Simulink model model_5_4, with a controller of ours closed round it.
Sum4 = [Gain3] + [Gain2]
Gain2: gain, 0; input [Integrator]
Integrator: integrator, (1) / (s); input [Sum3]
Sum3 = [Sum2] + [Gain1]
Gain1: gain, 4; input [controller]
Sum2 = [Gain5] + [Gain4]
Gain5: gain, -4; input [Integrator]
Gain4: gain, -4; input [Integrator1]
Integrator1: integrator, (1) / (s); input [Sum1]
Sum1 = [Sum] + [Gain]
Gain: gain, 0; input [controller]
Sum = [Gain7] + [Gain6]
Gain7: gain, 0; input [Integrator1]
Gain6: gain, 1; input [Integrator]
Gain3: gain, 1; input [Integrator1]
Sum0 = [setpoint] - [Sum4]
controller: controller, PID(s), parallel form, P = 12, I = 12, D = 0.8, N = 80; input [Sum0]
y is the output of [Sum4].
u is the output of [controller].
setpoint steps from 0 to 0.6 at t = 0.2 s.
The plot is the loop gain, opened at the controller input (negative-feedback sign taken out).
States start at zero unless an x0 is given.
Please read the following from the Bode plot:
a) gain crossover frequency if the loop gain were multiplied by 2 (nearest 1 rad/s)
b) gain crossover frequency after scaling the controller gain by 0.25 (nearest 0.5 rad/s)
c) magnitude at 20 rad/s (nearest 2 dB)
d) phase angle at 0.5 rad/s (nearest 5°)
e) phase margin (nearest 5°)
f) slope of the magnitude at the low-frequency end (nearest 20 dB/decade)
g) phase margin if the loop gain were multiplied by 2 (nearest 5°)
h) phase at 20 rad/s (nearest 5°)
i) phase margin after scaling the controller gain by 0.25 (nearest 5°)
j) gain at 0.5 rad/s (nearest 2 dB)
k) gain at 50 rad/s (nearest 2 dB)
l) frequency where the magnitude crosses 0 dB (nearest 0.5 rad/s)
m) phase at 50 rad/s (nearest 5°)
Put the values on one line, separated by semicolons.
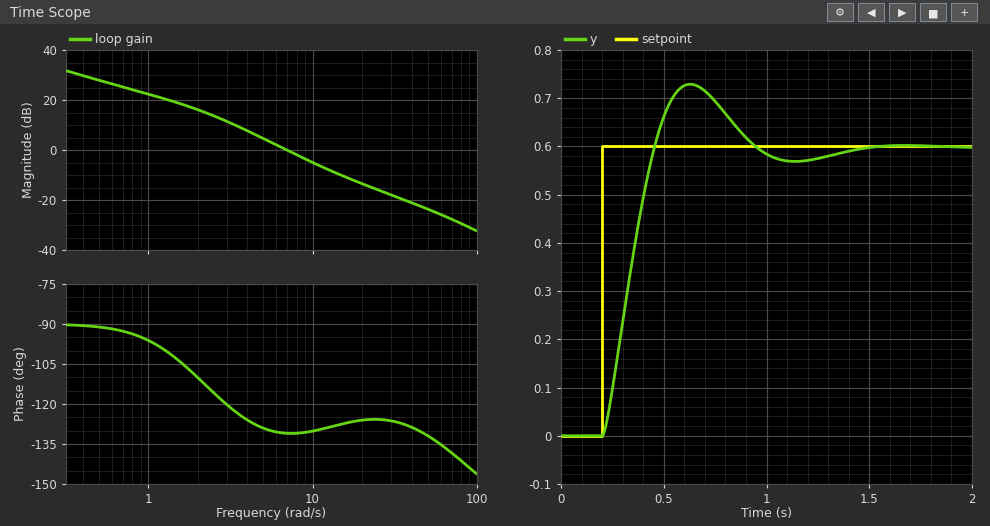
11 rad/s; 3.0 rad/s; -14 dB; -90°; 50°; -20 dB/decade; 50°; -125°; 60°; 28 dB; -24 dB; 7.0 rad/s; -130°
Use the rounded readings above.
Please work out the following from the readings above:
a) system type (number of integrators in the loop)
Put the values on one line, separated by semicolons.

1
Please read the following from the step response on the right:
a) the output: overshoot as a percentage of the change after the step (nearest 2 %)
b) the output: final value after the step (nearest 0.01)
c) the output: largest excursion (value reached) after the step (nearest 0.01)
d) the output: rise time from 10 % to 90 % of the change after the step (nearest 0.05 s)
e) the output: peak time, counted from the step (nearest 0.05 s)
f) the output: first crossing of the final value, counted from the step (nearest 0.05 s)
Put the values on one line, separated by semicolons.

22 %; 0.60; 0.73; 0.20 s; 0.45 s; 0.25 s
